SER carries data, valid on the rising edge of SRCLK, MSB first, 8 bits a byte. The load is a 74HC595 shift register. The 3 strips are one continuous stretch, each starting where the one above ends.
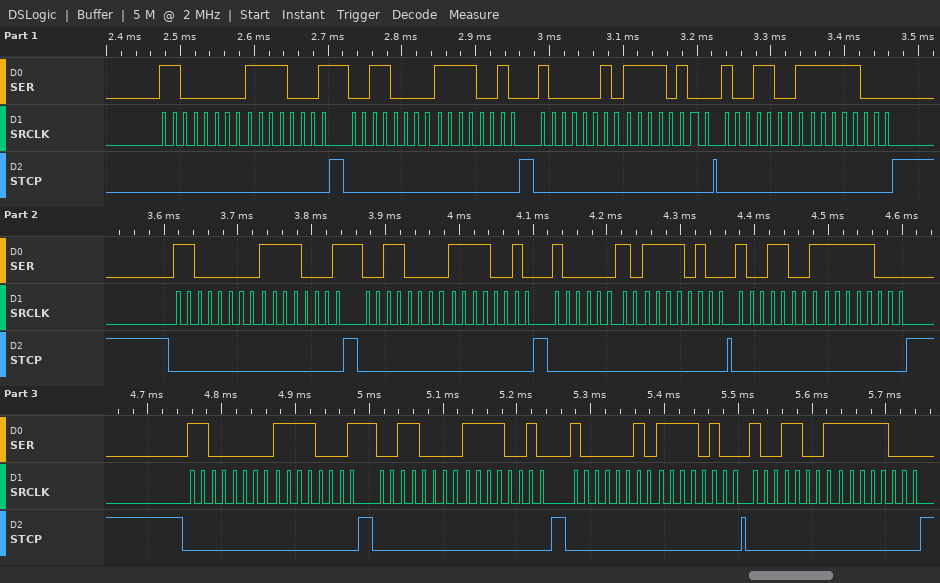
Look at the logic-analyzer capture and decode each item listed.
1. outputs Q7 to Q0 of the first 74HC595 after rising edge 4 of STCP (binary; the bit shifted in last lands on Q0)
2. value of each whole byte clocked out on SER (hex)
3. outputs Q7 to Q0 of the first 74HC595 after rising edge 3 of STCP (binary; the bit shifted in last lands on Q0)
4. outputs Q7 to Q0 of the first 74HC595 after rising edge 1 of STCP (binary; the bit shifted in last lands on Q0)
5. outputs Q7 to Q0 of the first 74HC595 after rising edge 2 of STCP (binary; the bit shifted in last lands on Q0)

11111000
C0 F1 30 F2 82 F4 99 F8 C0 F1 30 F2 82 F4 99 F8 C0 F1 30 F2 82 F4 99 F8
11110100
11110001
11110010
